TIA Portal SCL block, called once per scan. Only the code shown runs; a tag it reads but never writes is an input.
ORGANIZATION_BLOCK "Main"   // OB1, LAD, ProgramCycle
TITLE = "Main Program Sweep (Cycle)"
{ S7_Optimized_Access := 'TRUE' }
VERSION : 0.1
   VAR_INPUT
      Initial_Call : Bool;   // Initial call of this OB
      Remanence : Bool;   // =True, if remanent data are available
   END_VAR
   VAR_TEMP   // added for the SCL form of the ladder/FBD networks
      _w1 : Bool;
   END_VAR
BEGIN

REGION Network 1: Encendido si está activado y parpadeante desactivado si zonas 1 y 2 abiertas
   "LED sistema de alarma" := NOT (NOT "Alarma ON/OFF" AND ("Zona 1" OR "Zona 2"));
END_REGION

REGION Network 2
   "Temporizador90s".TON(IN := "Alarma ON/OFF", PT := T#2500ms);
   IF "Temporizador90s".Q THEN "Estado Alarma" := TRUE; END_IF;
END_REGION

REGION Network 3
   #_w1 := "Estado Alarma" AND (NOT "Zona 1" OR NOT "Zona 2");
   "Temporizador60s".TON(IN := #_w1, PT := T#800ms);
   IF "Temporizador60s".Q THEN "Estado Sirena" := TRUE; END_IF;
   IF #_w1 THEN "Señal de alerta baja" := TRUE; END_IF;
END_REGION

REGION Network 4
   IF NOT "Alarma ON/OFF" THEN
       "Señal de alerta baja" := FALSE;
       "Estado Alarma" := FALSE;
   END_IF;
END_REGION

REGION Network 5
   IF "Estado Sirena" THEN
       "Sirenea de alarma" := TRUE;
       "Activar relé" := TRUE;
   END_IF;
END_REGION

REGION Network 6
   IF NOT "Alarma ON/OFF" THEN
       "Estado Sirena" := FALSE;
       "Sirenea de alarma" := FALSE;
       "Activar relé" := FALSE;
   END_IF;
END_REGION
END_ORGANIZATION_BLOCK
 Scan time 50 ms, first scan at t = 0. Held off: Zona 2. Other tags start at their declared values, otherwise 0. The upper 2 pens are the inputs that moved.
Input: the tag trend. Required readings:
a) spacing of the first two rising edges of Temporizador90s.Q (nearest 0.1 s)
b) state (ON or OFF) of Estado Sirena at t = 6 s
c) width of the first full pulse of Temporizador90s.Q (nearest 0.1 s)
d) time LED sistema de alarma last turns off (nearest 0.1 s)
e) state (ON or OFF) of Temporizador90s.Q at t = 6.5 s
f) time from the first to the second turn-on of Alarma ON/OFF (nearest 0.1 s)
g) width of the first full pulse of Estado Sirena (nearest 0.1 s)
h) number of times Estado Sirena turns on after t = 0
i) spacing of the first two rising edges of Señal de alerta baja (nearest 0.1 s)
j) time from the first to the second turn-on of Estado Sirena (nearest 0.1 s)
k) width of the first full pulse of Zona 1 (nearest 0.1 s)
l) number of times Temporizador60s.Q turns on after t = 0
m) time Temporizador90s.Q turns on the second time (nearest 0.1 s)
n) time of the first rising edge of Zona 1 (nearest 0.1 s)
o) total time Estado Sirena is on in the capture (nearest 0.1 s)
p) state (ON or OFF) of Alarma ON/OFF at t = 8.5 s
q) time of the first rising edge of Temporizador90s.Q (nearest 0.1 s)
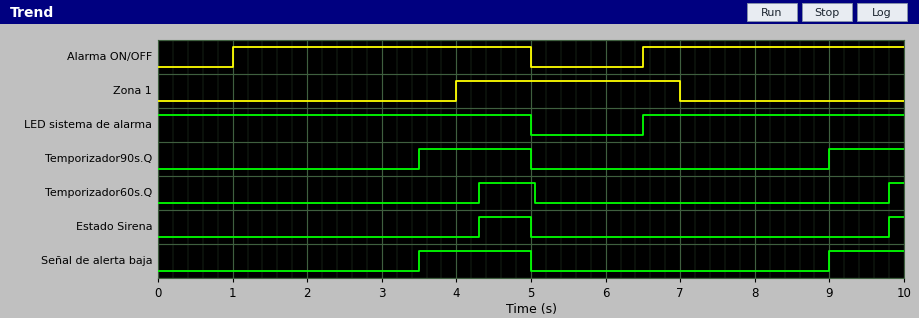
5.5 s
OFF
1.5 s
5.0 s
OFF
5.5 s
0.7 s
2
5.5 s
5.5 s
3.0 s
2
9.0 s
4.0 s
0.9 s
ON
3.5 s
